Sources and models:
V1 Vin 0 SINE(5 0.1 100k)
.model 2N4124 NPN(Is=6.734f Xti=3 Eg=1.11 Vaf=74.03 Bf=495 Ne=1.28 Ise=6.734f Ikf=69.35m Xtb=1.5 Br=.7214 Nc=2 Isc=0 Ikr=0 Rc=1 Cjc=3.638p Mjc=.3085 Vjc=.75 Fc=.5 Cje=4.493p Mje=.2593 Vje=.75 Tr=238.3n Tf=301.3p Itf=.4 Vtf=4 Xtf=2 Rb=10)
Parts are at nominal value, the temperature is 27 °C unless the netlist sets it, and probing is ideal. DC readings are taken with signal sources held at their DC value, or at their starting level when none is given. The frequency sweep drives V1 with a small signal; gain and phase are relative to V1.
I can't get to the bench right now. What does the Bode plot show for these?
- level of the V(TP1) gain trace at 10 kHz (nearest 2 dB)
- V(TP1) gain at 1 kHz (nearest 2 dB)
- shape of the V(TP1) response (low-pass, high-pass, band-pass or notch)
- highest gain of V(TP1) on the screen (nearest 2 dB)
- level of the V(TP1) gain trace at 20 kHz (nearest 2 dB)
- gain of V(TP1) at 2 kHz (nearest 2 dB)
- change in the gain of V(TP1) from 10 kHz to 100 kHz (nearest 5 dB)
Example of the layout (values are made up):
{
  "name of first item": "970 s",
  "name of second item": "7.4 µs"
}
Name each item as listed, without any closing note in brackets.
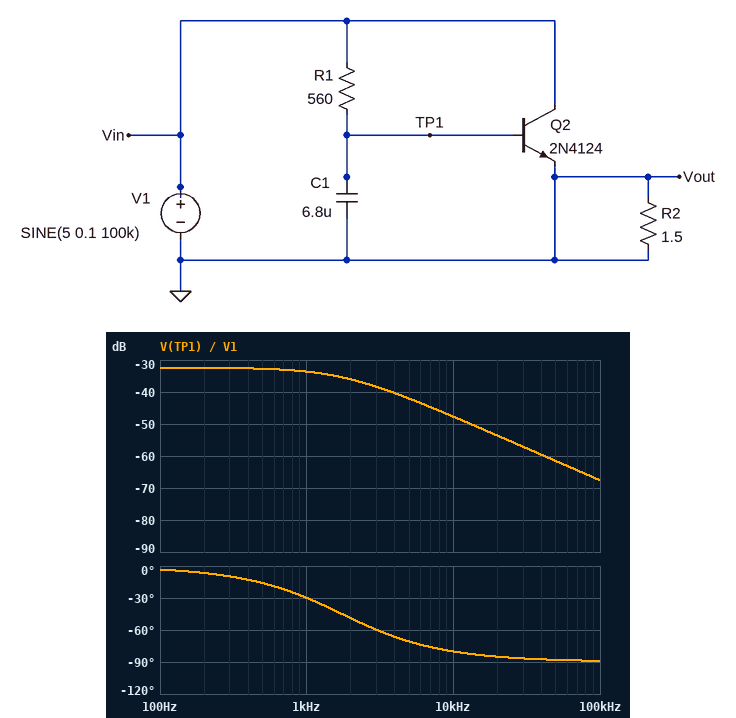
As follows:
{
  "level of the V(TP1) gain trace at 10 kHz": "-48 dB",
  "V(TP1) gain at 1 kHz": "-34 dB",
  "shape of the V(TP1) response": "low-pass",
  "highest gain of V(TP1) on the screen": "-32 dB",
  "level of the V(TP1) gain trace at 20 kHz": "-54 dB",
  "gain of V(TP1) at 2 kHz": "-36 dB",
  "change in the gain of V(TP1) from 10 kHz to 100 kHz": "-20 dB"
}
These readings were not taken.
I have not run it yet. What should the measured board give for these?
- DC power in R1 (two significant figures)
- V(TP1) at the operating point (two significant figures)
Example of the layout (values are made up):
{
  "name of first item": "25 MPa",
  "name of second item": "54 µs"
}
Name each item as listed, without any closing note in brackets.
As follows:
{
  "DC power in R1": "29 mW",
  "V(TP1) at the operating point": "940 mV"
}
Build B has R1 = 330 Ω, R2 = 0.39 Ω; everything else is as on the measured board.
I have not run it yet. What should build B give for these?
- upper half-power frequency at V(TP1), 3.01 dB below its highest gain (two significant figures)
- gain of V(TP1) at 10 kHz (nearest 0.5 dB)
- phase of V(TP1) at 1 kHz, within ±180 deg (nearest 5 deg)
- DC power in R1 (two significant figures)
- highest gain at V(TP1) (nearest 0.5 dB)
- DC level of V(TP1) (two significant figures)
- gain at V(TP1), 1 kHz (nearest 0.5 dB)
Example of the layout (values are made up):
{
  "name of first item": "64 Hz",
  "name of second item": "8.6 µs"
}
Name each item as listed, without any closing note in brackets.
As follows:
{
  "upper half-power frequency at V(TP1), 3.01 dB below its highest gain": "2.0 kHz",
  "gain of V(TP1) at 10 kHz": "-43.0 dB",
  "phase of V(TP1) at 1 kHz, within ±180 deg": "-25 deg",
  "DC power in R1": "48 mW",
  "highest gain at V(TP1)": "-29.0 dB",
  "DC level of V(TP1)": "1.0 V",
  "gain at V(TP1), 1 kHz": "-30.0 dB"
}
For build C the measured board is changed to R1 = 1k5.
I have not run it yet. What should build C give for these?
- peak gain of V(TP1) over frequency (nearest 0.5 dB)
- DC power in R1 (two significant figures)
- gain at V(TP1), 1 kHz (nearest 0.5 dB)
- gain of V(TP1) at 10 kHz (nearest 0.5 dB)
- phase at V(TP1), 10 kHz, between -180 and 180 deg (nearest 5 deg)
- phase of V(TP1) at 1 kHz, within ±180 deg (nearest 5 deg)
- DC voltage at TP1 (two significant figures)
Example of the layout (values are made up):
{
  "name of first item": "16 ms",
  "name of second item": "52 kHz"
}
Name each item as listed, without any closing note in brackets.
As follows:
{
  "peak gain of V(TP1) over frequency": "-37.5 dB",
  "DC power in R1": "11 mW",
  "gain at V(TP1), 1 kHz": "-40.0 dB",
  "gain of V(TP1) at 10 kHz": "-56.0 dB",
  "phase at V(TP1), 10 kHz, between -180 and 180 deg": "-85 deg",
  "phase of V(TP1) at 1 kHz, within ±180 deg": "-40 deg",
  "DC voltage at TP1": "870 mV"
}
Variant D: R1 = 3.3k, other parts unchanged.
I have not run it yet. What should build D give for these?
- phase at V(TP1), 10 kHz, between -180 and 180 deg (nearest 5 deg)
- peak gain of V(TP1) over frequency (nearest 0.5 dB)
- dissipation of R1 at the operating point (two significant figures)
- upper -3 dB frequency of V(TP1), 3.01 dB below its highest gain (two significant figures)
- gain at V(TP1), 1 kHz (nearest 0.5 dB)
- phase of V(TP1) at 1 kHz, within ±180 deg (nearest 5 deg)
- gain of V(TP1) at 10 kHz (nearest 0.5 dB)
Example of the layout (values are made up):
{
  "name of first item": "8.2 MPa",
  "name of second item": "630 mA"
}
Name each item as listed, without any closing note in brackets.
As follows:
{
  "phase at V(TP1), 10 kHz, between -180 and 180 deg": "-85 deg",
  "peak gain of V(TP1) over frequency": "-40.5 dB",
  "dissipation of R1 at the operating point": "5.3 mW",
  "upper -3 dB frequency of V(TP1), 3.01 dB below its highest gain": "740 Hz",
  "gain at V(TP1), 1 kHz": "-45.0 dB",
  "phase of V(TP1) at 1 kHz, within ±180 deg": "-55 deg",
  "gain of V(TP1) at 10 kHz": "-63.0 dB"
}
